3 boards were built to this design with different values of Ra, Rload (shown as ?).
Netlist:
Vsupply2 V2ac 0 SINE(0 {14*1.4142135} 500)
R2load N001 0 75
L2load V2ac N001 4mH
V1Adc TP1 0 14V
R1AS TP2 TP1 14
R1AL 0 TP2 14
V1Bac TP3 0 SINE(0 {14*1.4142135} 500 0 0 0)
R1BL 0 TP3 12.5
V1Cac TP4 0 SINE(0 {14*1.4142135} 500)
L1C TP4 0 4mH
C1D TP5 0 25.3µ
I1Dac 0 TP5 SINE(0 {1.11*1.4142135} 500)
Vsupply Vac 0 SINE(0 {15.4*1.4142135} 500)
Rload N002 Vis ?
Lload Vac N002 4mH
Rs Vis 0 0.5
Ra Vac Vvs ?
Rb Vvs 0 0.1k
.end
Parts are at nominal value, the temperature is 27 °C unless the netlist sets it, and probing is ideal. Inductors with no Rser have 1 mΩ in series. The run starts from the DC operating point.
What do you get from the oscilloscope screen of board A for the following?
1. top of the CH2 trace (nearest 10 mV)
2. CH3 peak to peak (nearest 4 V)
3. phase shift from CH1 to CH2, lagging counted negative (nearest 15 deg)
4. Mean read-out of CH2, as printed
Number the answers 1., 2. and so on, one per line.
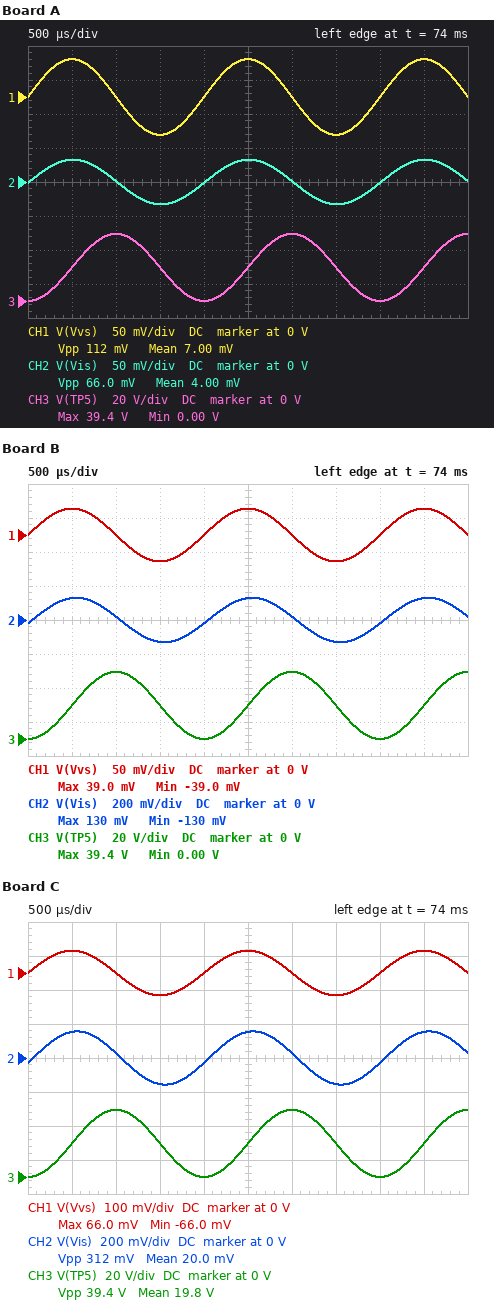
1. 30 mV
2. 40 V
3. 0 deg
4. 4.00 mV
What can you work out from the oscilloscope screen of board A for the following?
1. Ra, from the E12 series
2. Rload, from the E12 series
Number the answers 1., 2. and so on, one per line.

1. 39 kΩ
2. 330 Ω
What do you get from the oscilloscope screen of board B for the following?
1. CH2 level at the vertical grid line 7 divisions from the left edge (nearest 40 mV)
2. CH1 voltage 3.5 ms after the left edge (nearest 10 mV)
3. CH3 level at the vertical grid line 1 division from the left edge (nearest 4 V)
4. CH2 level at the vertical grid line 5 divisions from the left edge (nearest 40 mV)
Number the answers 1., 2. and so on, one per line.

1. -120 mV
2. -40 mV
3. 20 V
4. 120 mV
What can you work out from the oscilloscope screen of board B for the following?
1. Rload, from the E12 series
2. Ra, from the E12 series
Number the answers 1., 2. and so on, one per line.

1. 82 Ω
2. 56 kΩ
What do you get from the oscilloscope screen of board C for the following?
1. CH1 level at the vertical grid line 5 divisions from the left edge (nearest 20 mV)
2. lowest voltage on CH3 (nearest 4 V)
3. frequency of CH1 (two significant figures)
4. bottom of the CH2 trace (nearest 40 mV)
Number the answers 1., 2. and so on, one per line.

1. 60 mV
2. 0 V
3. 500 Hz
4. -160 mV
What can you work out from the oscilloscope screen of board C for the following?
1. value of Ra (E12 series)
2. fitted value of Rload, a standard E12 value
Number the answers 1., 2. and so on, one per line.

1. 33 kΩ
2. 68 Ω
